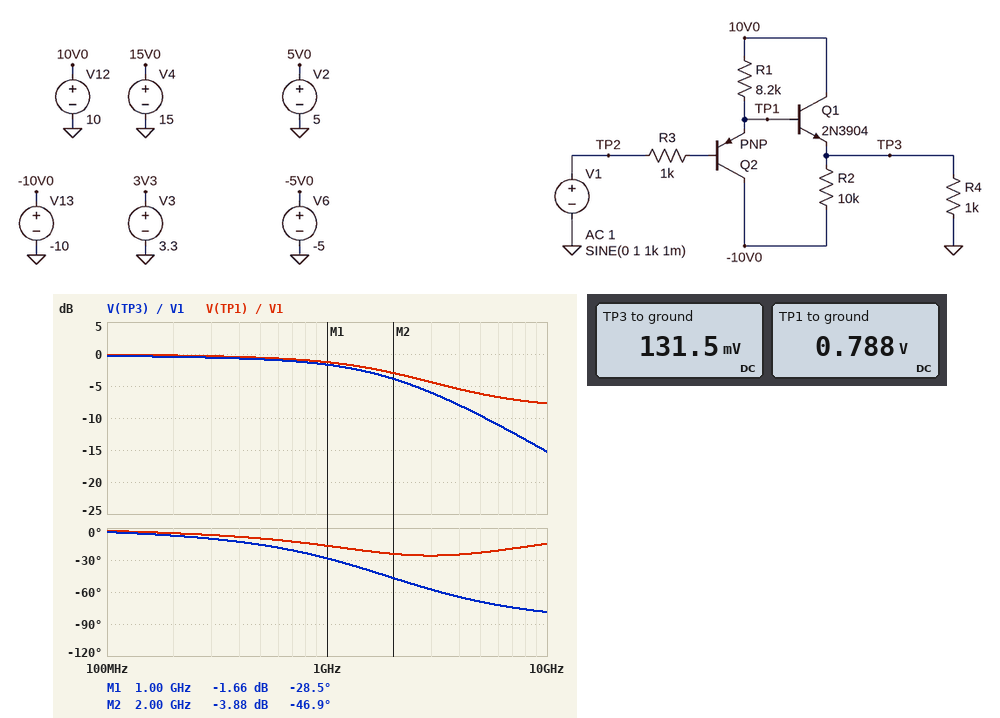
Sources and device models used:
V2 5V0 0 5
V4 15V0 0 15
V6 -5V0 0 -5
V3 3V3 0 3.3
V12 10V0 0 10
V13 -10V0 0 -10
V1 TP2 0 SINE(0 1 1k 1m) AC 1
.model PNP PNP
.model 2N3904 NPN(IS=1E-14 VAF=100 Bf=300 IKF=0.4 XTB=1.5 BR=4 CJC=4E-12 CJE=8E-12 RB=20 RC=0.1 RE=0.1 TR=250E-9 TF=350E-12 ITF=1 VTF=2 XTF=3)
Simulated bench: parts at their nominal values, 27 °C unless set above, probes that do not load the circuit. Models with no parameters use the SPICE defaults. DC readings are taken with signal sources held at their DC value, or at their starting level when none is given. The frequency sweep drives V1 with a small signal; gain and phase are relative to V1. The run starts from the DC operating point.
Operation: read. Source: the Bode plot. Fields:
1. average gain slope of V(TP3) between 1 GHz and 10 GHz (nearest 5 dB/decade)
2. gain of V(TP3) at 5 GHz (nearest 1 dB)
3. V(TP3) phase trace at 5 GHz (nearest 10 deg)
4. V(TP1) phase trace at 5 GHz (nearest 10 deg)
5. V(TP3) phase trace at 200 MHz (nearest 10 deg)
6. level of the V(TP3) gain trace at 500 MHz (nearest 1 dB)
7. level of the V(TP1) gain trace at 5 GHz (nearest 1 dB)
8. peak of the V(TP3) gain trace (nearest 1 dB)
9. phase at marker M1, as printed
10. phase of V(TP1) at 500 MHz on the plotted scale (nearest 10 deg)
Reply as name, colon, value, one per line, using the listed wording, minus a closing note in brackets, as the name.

average gain slope of V(TP3) between 1 GHz and 10 GHz: -15 dB/decade
gain of V(TP3) at 5 GHz: -10 dB
V(TP3) phase trace at 5 GHz: -70 deg
V(TP1) phase trace at 5 GHz: -20 deg
V(TP3) phase trace at 200 MHz: -10 deg
level of the V(TP3) gain trace at 500 MHz: -1 dB
level of the V(TP1) gain trace at 5 GHz: -6 dB
peak of the V(TP3) gain trace: 0 dB
phase at marker M1, as printed: -28.5 deg
phase of V(TP1) at 500 MHz on the plotted scale: -10 deg
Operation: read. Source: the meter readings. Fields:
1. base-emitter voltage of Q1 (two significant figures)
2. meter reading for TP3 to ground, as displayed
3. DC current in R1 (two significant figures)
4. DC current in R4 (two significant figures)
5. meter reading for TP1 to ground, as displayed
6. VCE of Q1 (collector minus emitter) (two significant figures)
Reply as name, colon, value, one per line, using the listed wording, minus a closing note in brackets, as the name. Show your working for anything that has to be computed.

base-emitter voltage of Q1: 788 mV - 131.5 mV = 660 mV
meter reading for TP3 to ground, as displayed: 131.5 mV
DC current in R1: (10 V - 788 mV) / 8.2 kΩ = 1.1 mA
DC current in R4: (131.5 mV) / 1 kΩ = 130 µA
meter reading for TP1 to ground, as displayed: 0.788 V
VCE of Q1 (collector minus emitter): 10 V - 131.5 mV = 9.9 V
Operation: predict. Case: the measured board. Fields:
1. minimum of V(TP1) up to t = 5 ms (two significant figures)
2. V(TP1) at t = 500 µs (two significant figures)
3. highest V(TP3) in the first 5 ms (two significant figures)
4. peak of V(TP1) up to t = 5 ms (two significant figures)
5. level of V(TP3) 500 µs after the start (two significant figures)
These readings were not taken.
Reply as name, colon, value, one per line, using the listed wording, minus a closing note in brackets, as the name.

minimum of V(TP1) up to t = 5 ms: -210 mV
V(TP1) at t = 500 µs: 790 mV
highest V(TP3) in the first 5 ms: 1.1 V
peak of V(TP1) up to t = 5 ms: 1.8 V
level of V(TP3) 500 µs after the start: 130 mV
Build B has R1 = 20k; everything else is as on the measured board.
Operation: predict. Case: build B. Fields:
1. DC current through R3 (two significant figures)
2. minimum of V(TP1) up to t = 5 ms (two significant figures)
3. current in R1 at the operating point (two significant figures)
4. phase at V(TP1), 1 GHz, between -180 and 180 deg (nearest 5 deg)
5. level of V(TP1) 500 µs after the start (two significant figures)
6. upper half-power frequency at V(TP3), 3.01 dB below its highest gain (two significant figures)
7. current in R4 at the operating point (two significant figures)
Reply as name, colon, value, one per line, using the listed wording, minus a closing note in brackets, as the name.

DC current through R3: 4.5 µA
minimum of V(TP1) up to t = 5 ms: -240 mV
current in R1 at the operating point: 460 µA
phase at V(TP1), 1 GHz, between -180 and 180 deg: -30 deg
level of V(TP1) 500 µs after the start: 760 mV
upper half-power frequency at V(TP3), 3.01 dB below its highest gain: 1.0 GHz
current in R4 at the operating point: 100 µA
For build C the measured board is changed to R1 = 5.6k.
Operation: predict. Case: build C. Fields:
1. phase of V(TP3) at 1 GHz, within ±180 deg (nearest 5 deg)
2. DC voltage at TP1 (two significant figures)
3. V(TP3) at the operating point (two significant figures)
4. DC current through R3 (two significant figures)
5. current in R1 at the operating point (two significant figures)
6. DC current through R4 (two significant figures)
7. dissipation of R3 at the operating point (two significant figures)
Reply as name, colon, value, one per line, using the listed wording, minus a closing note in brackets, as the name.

phase of V(TP3) at 1 GHz, within ±180 deg: -25 deg
DC voltage at TP1: 800 mV
V(TP3) at the operating point: 150 mV
DC current through R3: 16 µA
current in R1 at the operating point: 1.6 mA
DC current through R4: 150 µA
dissipation of R3 at the operating point: 260 nW
